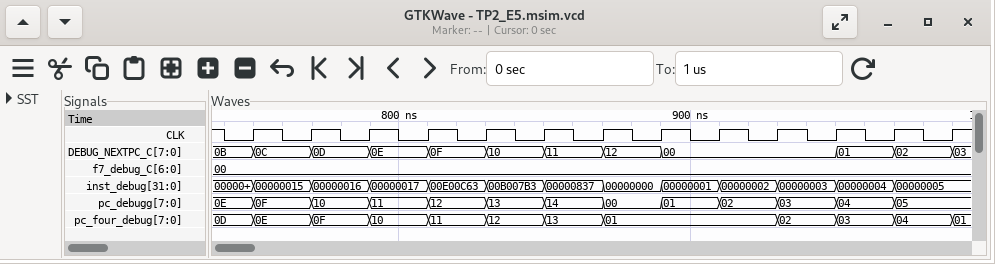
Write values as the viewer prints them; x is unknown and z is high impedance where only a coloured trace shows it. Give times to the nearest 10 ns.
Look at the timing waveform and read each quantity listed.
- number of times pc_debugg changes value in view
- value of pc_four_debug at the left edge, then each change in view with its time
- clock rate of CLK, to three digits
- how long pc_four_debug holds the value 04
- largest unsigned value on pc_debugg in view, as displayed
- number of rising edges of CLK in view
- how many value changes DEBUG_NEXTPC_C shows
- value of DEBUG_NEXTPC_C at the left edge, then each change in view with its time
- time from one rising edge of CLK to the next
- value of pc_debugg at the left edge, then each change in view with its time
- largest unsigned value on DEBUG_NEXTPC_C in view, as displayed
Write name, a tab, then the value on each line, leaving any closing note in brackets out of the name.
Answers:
number of times pc_debugg changes value in view	12
value of pc_four_debug at the left edge, then each change in view with its time	0D, 0E at 750 ns, 0F at 770 ns, 10 at 790 ns, 11 at 810 ns, 12 at 830 ns, 13 at 850 ns, 01 at 870 ns, 02 at 930 ns, 03 at 950 ns, 04 at 970 ns, 01 at 990 ns
clock rate of CLK, to three digits	50.0 MHz
how long pc_four_debug holds the value 04	20 ns
largest unsigned value on pc_debugg in view, as displayed	14
number of rising edges of CLK in view	13
how many value changes DEBUG_NEXTPC_C shows	11
value of DEBUG_NEXTPC_C at the left edge, then each change in view with its time	0B, 0C at 750 ns, 0D at 770 ns, 0E at 790 ns, 0F at 810 ns, 10 at 830 ns, 11 at 850 ns, 12 at 870 ns, 00 at 890 ns, 01 at 950 ns, 02 at 970 ns, 03 at 990 ns
time from one rising edge of CLK to the next	20 ns
value of pc_debugg at the left edge, then each change in view with its time	0E, 0F at 750 ns, 10 at 770 ns, 11 at 790 ns, 12 at 810 ns, 13 at 830 ns, 14 at 850 ns, 00 at 870 ns, 01 at 890 ns, 02 at 910 ns, 03 at 930 ns, 04 at 950 ns, 05 at 970 ns
largest unsigned value on DEBUG_NEXTPC_C in view, as displayed	12
